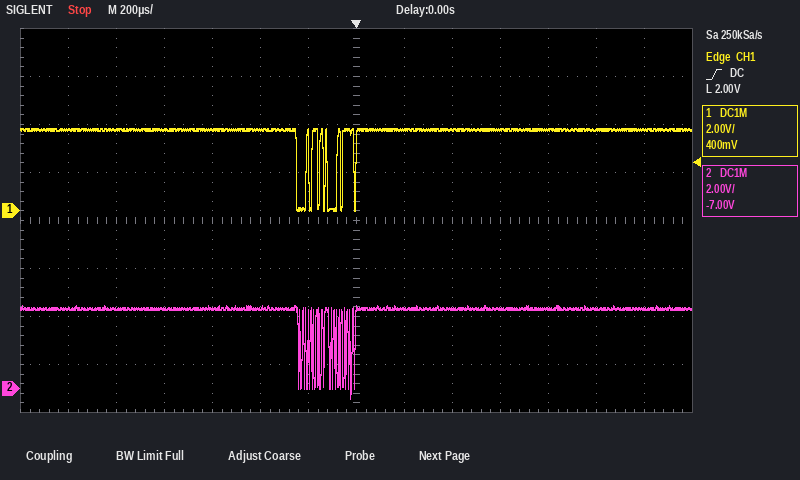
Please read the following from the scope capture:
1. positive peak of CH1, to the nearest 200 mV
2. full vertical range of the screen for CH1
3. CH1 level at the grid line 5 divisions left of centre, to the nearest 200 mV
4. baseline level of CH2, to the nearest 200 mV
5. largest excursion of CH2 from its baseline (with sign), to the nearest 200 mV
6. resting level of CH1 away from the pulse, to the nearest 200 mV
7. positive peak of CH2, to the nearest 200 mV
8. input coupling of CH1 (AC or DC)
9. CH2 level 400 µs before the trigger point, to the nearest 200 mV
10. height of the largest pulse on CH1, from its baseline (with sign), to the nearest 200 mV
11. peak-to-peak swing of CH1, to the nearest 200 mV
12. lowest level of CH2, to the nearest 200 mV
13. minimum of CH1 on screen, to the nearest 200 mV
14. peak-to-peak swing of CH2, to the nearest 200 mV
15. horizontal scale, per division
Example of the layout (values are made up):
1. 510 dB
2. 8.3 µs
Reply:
1. 3.4 V
2. 16 V
3. 3.4 V
4. 3.4 V
5. -3.8 V
6. 3.4 V
7. 3.4 V
8. DC
9. 3.4 V
10. -3.4 V
11. 3.4 V
12. -400 mV
13. 0.0 V
14. 3.8 V
15. 200 µs
